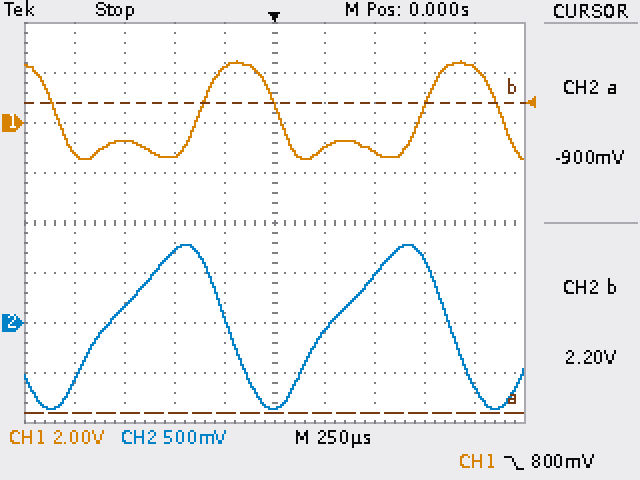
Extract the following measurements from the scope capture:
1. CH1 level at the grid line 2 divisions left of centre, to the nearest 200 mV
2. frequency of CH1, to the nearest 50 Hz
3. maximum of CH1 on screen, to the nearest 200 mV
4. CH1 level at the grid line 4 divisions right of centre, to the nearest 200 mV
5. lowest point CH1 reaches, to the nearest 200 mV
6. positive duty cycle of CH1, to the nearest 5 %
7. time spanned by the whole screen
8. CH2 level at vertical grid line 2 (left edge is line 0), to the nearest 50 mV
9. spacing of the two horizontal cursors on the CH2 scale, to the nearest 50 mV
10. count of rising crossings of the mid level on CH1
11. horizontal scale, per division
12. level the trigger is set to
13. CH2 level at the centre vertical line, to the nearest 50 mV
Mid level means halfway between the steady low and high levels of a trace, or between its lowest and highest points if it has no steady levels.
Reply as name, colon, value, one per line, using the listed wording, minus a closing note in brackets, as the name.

CH1 level at the grid line 2 divisions left of centre, to the nearest 200 mV: -1.4 V
frequency of CH1, to the nearest 50 Hz: 900 Hz
maximum of CH1 on screen, to the nearest 200 mV: 2.4 V
CH1 level at the grid line 4 divisions right of centre, to the nearest 200 mV: 2.2 V
lowest point CH1 reaches, to the nearest 200 mV: -1.4 V
positive duty cycle of CH1, to the nearest 5 %: 35 %
time spanned by the whole screen: 2.5 ms
CH2 level at vertical grid line 2 (left edge is line 0), to the nearest 50 mV: 150 mV
spacing of the two horizontal cursors on the CH2 scale, to the nearest 50 mV: 3.10 V
count of rising crossings of the mid level on CH1: 2
horizontal scale, per division: 250 µs
level the trigger is set to: 800 mV
CH2 level at the centre vertical line, to the nearest 50 mV: -850 mV
